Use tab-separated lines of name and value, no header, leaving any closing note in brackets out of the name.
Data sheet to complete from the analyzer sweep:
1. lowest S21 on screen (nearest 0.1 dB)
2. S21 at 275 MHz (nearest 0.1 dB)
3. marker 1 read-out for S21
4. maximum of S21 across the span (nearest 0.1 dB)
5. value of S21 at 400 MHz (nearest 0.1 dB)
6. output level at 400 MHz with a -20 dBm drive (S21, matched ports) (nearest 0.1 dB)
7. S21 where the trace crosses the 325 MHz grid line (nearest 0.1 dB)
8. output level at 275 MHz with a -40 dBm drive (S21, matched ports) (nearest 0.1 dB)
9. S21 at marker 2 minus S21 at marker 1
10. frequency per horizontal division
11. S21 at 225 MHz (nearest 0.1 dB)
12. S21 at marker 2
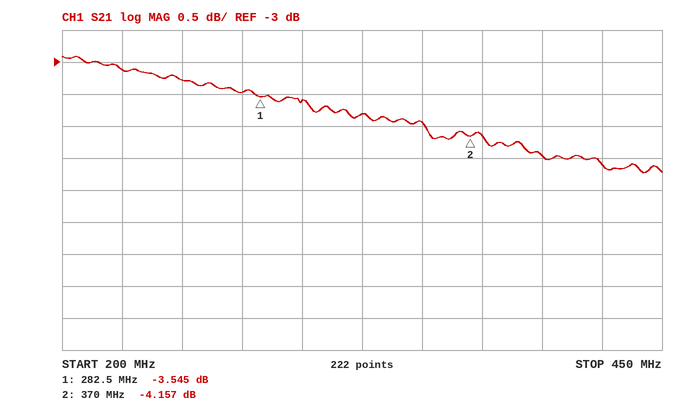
lowest S21 on screen	-4.7 dB
S21 at 275 MHz	-3.5 dB
marker 1 read-out for S21	-3.545 dB
maximum of S21 across the span	-2.9 dB
value of S21 at 400 MHz	-4.5 dB
output level at 400 MHz with a -20 dBm drive (S21, matched ports)	-24.5 dBm
S21 where the trace crosses the 325 MHz grid line	-3.8 dB
output level at 275 MHz with a -40 dBm drive (S21, matched ports)	-43.5 dBm
S21 at marker 2 minus S21 at marker 1	-0.612 dB
frequency per horizontal division	25 MHz
S21 at 225 MHz	-3.1 dB
S21 at marker 2	-4.157 dB
